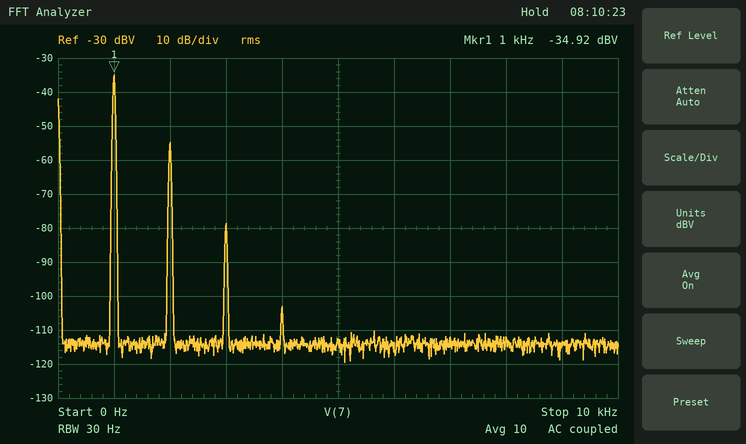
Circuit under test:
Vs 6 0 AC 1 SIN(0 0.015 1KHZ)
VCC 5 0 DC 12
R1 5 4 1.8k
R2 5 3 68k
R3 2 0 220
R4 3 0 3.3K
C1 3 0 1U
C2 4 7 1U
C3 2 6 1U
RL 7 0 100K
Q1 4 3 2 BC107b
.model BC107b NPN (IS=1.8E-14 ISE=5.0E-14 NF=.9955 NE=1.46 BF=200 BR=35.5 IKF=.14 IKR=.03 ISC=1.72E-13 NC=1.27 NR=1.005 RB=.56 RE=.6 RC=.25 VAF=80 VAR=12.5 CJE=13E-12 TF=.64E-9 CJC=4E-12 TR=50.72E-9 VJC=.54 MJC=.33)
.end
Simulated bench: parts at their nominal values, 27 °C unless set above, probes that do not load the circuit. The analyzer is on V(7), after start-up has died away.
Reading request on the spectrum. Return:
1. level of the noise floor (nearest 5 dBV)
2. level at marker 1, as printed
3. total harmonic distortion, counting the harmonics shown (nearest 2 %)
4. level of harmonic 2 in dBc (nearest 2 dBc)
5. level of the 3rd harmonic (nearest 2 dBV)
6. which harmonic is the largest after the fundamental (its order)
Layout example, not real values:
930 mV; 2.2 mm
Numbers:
-115 dBV; -34.92 dBV; 10 %; -20 dBc; -78 dBV; 2
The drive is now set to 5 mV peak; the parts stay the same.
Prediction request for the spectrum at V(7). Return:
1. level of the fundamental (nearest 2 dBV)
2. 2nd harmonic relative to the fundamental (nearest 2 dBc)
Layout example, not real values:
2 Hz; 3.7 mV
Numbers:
-44 dBV; -30 dBc
